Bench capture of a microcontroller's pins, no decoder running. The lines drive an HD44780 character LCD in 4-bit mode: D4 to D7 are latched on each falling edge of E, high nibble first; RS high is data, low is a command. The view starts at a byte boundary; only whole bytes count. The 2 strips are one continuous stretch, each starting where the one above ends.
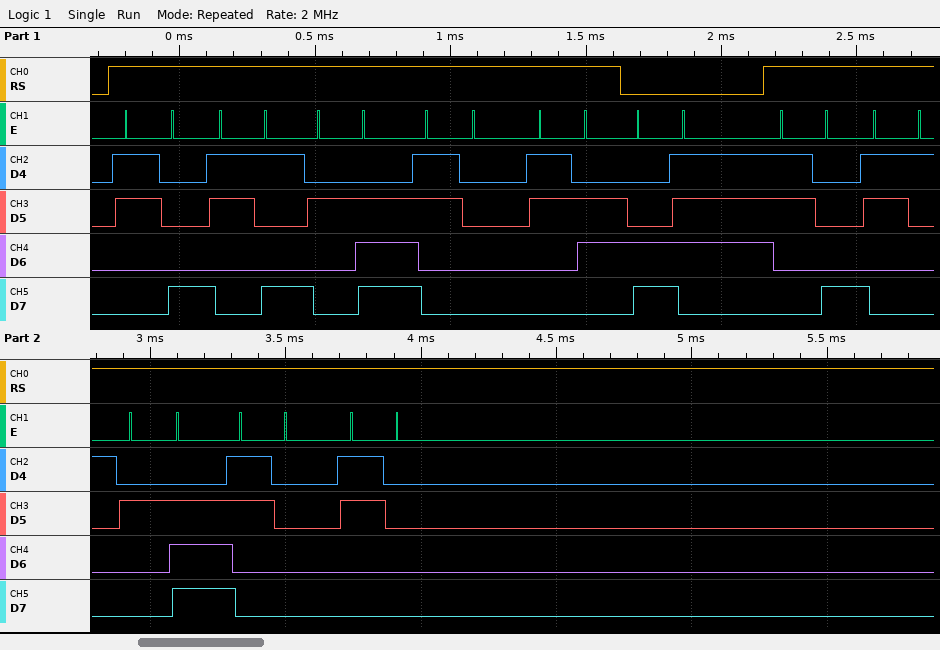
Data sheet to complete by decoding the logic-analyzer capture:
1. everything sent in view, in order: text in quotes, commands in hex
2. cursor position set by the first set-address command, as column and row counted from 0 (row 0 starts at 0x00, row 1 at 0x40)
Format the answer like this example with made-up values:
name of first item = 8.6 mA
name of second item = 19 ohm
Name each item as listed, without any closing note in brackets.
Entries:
everything sent in view, in order: text in quotes, commands in hex = "89.06" 0xC7 "81.00"
cursor position set by the first set-address command, as column and row counted from 0 = column 7, row 1
